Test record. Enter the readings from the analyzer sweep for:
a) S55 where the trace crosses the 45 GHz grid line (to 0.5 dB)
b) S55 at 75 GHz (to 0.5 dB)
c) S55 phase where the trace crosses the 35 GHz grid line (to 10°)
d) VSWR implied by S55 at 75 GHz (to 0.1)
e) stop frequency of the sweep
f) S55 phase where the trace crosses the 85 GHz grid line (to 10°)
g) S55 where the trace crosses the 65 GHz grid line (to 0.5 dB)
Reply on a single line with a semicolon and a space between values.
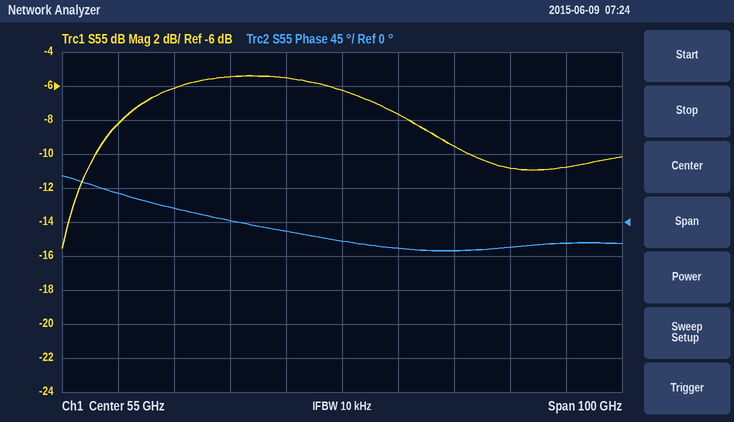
-5.5 dB; -9.5 dB; 0°; 2.0; 105 GHz; -30°; -7.5 dB
